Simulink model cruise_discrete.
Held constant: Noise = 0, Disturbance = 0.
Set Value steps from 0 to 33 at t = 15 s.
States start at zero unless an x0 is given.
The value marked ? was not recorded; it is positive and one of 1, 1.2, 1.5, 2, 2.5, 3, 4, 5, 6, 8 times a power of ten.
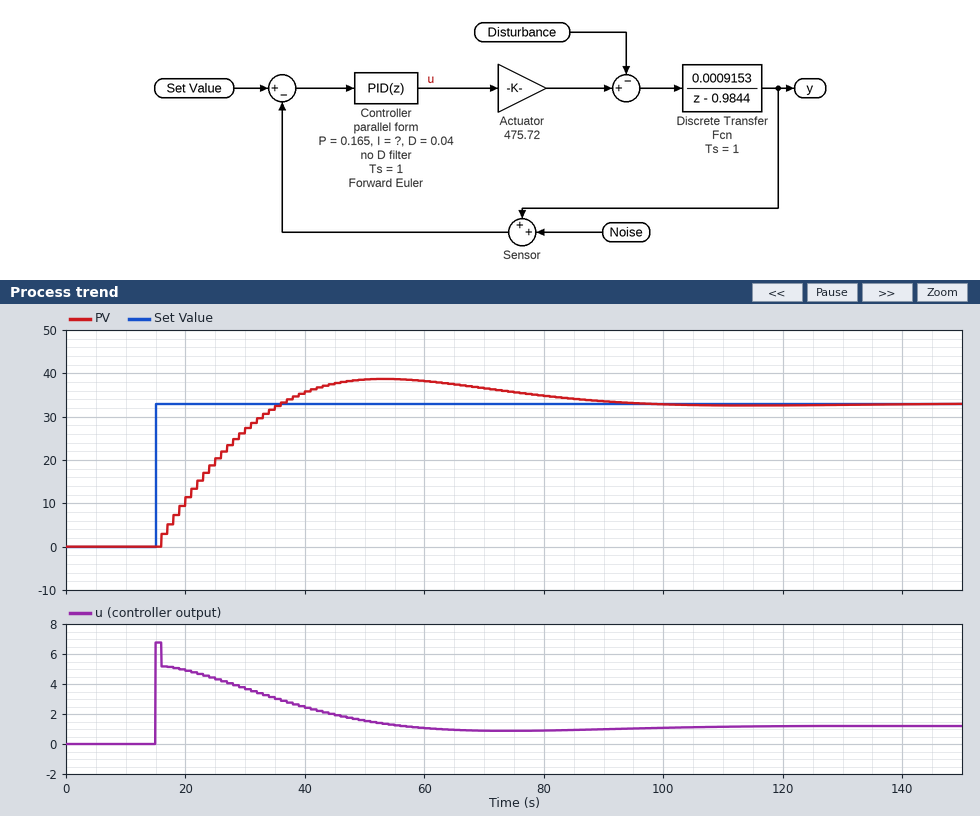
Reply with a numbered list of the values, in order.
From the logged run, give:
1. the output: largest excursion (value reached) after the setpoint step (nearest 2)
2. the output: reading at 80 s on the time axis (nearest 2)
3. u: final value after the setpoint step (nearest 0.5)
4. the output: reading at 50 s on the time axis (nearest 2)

1. 38
2. 34
3. 1.0
4. 38
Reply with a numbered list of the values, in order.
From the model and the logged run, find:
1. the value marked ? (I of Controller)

1. 0.01
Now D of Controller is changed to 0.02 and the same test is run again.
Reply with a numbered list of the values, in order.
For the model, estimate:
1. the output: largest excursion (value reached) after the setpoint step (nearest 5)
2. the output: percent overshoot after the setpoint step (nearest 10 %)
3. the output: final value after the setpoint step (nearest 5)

1. 40
2. 20 %
3. 35
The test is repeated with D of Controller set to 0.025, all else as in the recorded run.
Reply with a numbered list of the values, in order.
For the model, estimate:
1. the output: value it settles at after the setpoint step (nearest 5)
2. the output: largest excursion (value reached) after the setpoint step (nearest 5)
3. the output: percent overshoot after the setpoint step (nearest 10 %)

1. 35
2. 40
3. 20 %
